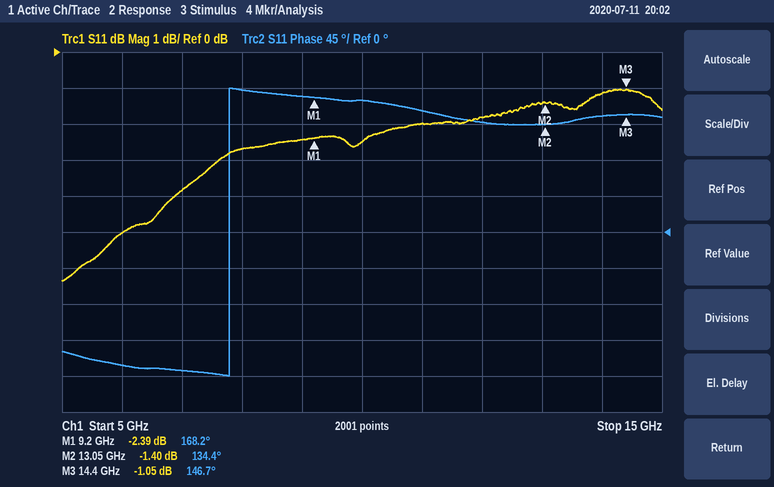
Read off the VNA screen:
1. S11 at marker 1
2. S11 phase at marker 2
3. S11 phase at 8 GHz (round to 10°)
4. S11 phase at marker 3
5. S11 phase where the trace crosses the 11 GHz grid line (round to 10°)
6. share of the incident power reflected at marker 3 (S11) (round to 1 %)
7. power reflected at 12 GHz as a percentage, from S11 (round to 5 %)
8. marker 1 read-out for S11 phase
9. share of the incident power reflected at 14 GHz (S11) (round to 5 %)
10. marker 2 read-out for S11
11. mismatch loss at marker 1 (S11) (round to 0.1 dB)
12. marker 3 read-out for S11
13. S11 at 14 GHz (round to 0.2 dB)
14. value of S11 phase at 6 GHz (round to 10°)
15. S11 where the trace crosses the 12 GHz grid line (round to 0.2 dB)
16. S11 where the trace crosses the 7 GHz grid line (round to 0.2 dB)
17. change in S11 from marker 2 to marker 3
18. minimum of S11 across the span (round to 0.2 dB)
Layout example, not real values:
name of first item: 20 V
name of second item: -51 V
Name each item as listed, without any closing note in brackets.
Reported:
S11 at marker 1: -2.39 dB
S11 phase at marker 2: 134.4°
S11 phase at 8 GHz: 180°
S11 phase at marker 3: 146.7°
S11 phase where the trace crosses the 11 GHz grid line: 150°
share of the incident power reflected at marker 3 (S11): 79 %
power reflected at 12 GHz as a percentage, from S11: 65 %
marker 1 read-out for S11 phase: 168.2°
share of the incident power reflected at 14 GHz (S11): 75 %
marker 2 read-out for S11: -1.40 dB
mismatch loss at marker 1 (S11): 3.7 dB
marker 3 read-out for S11: -1.05 dB
S11 at 14 GHz: -1.2 dB
value of S11 phase at 6 GHz: -170°
S11 where the trace crosses the 12 GHz grid line: -1.8 dB
S11 where the trace crosses the 7 GHz grid line: -3.8 dB
change in S11 from marker 2 to marker 3: 0.35 dB
minimum of S11 across the span: -6.4 dB
